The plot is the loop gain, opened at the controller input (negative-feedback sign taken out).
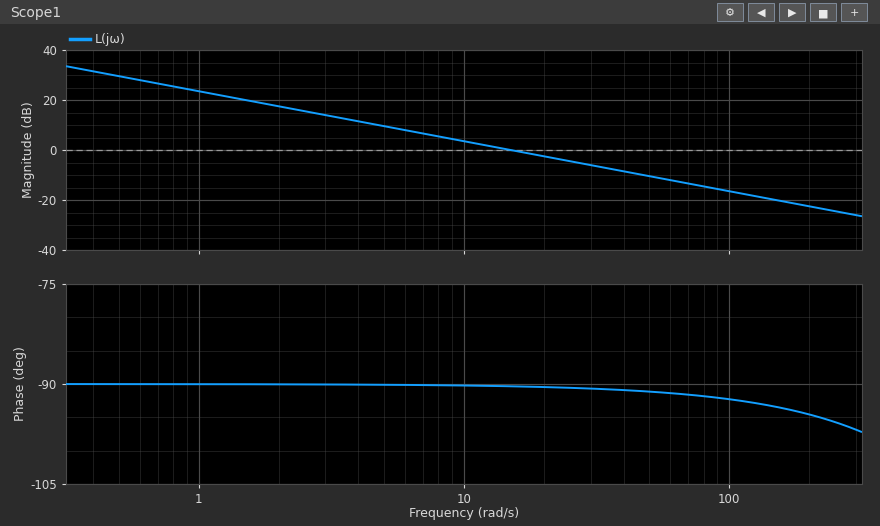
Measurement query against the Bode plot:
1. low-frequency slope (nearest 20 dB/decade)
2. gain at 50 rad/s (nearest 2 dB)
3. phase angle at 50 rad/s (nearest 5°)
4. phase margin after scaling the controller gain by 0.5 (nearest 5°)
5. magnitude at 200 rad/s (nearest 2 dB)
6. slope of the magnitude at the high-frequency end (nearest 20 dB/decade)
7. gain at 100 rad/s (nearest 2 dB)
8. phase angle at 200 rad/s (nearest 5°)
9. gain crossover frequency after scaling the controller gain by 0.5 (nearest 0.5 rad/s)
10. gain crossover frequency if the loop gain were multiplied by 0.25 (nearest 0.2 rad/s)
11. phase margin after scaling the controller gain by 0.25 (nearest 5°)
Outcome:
-20 dB/decade
-10 dB
-90°
90°
-22 dB
-20 dB/decade
-16 dB
-95°
7.5 rad/s
3.8 rad/s
90°
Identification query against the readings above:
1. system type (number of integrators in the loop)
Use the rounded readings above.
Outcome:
1
